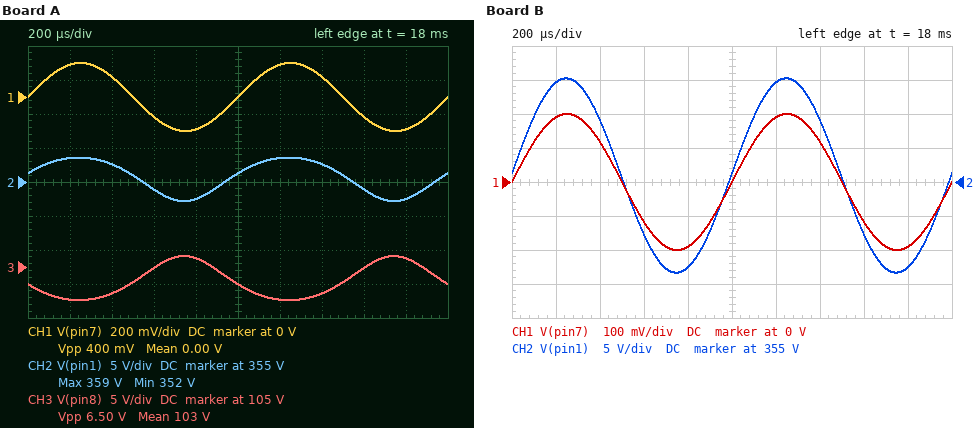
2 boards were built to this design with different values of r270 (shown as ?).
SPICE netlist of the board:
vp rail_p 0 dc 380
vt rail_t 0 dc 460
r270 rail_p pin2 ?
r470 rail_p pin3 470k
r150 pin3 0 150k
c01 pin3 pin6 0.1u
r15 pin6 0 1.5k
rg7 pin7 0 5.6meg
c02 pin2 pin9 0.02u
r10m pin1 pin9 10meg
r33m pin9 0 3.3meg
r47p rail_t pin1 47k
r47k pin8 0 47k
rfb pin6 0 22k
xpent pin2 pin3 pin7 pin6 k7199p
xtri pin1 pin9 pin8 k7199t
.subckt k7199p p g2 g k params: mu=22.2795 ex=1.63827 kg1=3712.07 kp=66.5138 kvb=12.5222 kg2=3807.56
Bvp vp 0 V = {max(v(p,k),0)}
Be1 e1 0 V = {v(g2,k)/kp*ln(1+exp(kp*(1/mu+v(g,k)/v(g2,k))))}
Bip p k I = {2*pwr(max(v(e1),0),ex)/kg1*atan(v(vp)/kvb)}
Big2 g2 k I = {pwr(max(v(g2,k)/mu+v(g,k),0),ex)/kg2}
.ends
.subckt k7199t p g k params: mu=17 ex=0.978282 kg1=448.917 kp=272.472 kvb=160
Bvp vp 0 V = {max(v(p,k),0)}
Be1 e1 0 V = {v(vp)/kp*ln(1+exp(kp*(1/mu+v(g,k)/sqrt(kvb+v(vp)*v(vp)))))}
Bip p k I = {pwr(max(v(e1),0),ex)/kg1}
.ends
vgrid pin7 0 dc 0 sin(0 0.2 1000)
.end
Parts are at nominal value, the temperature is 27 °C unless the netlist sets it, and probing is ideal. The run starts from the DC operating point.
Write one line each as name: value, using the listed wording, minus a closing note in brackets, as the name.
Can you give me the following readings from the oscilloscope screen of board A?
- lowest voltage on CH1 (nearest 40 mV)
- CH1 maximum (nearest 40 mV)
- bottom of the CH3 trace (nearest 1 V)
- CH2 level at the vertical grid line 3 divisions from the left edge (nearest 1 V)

lowest voltage on CH1: -200 mV
CH1 maximum: 200 mV
bottom of the CH3 trace: 100 V
CH2 level at the vertical grid line 3 divisions from the left edge: 354 V
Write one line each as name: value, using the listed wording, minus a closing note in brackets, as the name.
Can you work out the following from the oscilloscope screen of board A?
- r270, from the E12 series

r270, from the E12 series: 560 kΩ
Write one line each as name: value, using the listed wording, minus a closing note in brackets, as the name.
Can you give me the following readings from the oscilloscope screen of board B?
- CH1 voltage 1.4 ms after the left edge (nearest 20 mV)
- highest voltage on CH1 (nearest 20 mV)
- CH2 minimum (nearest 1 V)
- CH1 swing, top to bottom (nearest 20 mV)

CH1 voltage 1.4 ms after the left edge: 120 mV
highest voltage on CH1: 200 mV
CH2 minimum: 342 V
CH1 swing, top to bottom: 400 mV
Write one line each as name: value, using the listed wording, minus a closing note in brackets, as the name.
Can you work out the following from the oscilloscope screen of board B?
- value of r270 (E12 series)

value of r270: 220 kΩ
